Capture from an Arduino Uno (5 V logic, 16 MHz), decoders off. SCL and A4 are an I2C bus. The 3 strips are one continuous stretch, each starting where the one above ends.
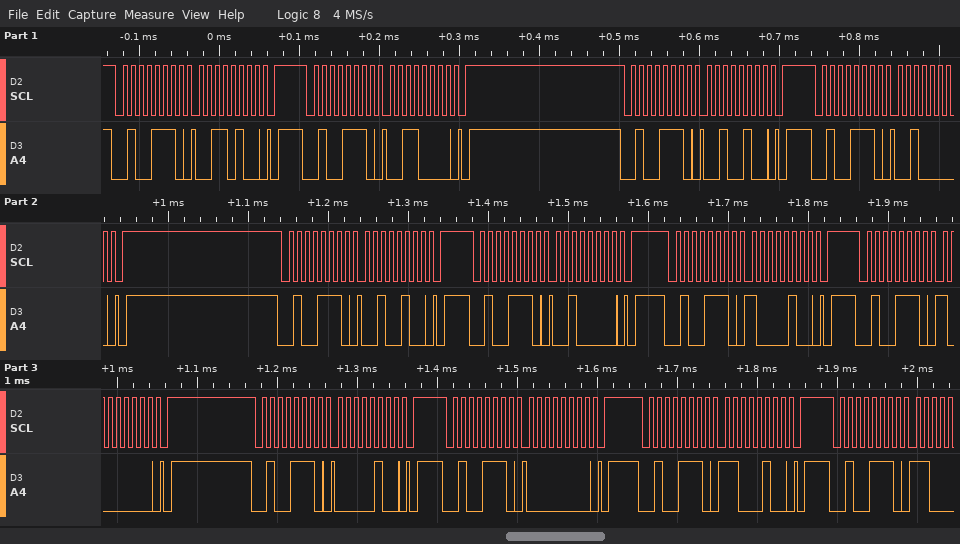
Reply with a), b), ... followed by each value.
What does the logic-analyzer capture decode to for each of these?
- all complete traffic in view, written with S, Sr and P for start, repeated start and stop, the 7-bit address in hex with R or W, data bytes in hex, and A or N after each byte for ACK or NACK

a) S 27W A 34 A P S 27W A 30 A P S 27W A 24 A P S 27W A 20 A P S 27W A 24 A P S 27W A 20 A P S 27W A 84 A P S 27W A 80 A P S 27W A 04 A P S 27W A 00 A P S 27W A C4 A P S 27W A
